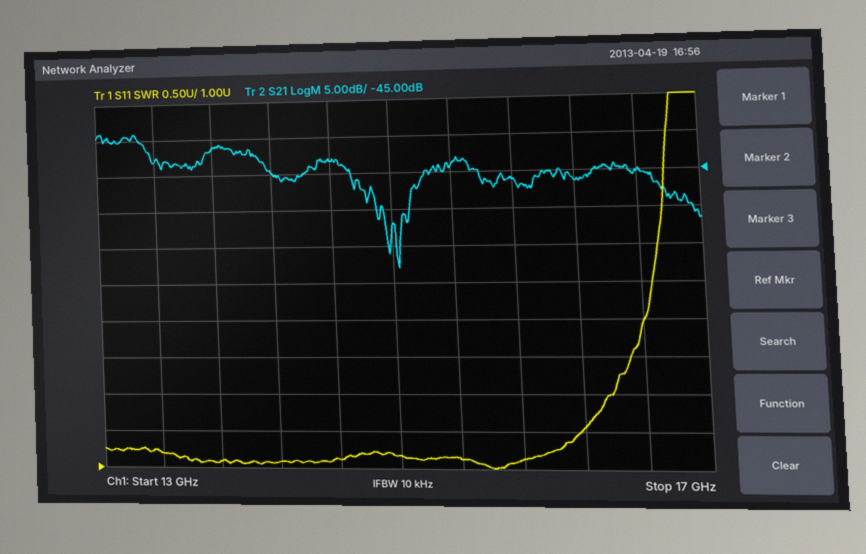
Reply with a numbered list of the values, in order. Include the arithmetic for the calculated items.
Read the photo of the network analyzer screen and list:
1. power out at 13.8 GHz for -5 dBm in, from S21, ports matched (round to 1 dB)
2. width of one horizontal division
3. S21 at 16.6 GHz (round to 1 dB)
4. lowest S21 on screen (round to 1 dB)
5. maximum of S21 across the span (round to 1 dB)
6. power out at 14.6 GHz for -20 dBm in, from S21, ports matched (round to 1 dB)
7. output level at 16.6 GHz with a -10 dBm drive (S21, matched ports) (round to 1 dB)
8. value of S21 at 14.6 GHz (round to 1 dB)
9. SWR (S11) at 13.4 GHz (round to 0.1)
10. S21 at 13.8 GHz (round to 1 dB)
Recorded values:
1. -5 dBm + (-41 dB) = -46 dBm
2. 400 MHz
3. -45 dB
4. -58 dB
5. -39 dB
6. -20 dBm + (-43 dB) = -63 dBm
7. -10 dBm + (-45 dB) = -55 dBm
8. -43 dB
9. 1.2
10. -41 dB
